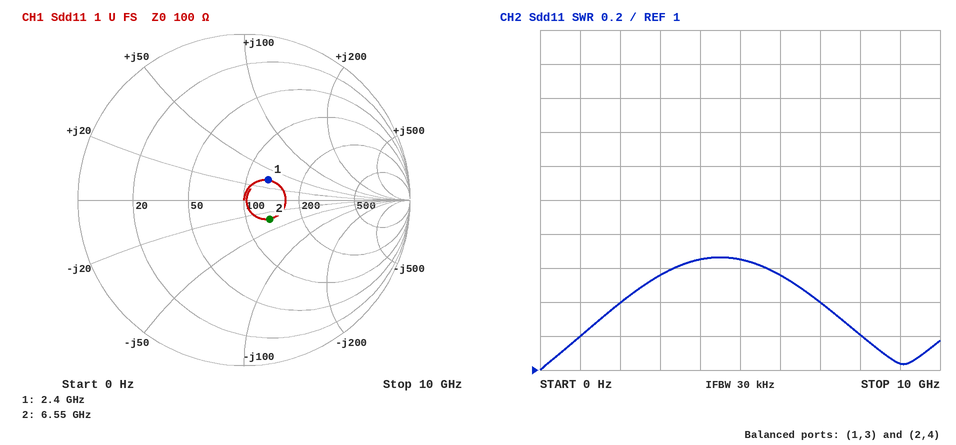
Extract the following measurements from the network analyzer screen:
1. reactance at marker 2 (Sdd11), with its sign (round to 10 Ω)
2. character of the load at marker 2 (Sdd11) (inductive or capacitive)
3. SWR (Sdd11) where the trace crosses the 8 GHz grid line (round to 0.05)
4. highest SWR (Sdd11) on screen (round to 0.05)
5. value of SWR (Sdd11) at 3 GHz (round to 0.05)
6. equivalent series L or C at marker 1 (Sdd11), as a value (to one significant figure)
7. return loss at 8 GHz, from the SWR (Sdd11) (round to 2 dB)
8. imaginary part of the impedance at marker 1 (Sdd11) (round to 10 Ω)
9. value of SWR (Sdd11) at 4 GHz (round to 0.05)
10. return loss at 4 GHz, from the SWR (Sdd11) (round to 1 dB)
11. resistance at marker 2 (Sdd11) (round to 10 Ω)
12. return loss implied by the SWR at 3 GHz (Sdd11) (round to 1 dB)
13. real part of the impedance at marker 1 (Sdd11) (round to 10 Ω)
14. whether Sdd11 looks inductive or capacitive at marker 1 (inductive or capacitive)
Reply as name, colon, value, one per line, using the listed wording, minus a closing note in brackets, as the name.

reactance at marker 2 (Sdd11), with its sign: -30 Ω
character of the load at marker 2 (Sdd11): capacitive
SWR (Sdd11) where the trace crosses the 8 GHz grid line: 1.20
highest SWR (Sdd11) on screen: 1.65
value of SWR (Sdd11) at 3 GHz: 1.55
equivalent series L or C at marker 1 (Sdd11), as a value: 2 nH
return loss at 8 GHz, from the SWR (Sdd11): 20 dB
imaginary part of the impedance at marker 1 (Sdd11): +30 Ω
value of SWR (Sdd11) at 4 GHz: 1.65
return loss at 4 GHz, from the SWR (Sdd11): 12 dB
resistance at marker 2 (Sdd11): 130 Ω
return loss implied by the SWR at 3 GHz (Sdd11): 13 dB
real part of the impedance at marker 1 (Sdd11): 130 Ω
whether Sdd11 looks inductive or capacitive at marker 1: inductive
